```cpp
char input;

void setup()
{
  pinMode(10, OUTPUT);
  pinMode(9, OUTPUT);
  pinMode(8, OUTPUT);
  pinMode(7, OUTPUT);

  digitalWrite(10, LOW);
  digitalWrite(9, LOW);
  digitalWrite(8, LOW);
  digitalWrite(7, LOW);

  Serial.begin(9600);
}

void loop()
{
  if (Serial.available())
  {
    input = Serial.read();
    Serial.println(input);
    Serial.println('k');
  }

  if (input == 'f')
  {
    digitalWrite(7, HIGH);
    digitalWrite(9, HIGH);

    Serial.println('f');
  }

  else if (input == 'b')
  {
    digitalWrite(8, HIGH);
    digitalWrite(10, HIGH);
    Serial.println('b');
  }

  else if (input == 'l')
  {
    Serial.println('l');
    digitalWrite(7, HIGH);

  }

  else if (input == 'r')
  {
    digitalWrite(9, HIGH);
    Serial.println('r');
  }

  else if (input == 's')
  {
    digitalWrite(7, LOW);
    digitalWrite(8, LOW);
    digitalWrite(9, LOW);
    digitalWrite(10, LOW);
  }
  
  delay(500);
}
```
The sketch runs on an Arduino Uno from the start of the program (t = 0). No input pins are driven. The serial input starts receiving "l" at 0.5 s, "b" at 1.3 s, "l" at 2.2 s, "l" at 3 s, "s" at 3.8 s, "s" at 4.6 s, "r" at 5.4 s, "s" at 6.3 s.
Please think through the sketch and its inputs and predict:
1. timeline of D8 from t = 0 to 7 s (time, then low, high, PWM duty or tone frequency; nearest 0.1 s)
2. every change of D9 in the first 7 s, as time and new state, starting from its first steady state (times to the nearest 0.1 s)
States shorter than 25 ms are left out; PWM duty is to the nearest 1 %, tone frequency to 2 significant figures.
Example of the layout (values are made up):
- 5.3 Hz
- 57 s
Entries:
- 0 s low; 1.5 s high; 4 s low
- 0 s low; 5.5 s high; 6.5 s low
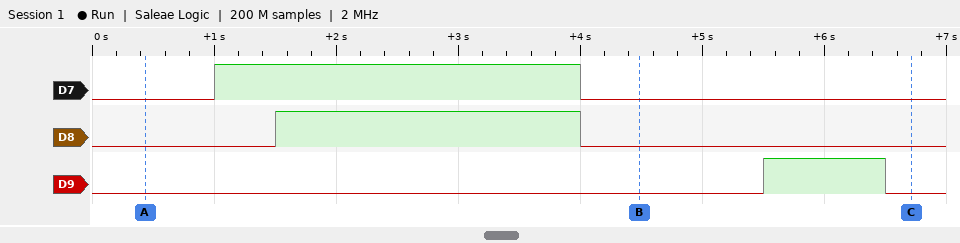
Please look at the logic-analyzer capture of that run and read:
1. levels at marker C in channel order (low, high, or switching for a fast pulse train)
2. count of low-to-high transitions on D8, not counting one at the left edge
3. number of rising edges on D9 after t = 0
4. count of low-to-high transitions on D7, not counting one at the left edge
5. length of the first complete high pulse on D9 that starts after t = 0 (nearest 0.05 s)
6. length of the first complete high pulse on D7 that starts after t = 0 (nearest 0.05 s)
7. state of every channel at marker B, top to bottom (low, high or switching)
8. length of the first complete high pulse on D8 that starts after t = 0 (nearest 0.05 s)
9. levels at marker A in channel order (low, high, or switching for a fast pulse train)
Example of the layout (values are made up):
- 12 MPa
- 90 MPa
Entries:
- D7 low, D8 low, D9 low
- 1
- 1
- 1
- 1.00 s
- 3.00 s
- D7 low, D8 low, D9 low
- 2.50 s
- D7 low, D8 low, D9 low
